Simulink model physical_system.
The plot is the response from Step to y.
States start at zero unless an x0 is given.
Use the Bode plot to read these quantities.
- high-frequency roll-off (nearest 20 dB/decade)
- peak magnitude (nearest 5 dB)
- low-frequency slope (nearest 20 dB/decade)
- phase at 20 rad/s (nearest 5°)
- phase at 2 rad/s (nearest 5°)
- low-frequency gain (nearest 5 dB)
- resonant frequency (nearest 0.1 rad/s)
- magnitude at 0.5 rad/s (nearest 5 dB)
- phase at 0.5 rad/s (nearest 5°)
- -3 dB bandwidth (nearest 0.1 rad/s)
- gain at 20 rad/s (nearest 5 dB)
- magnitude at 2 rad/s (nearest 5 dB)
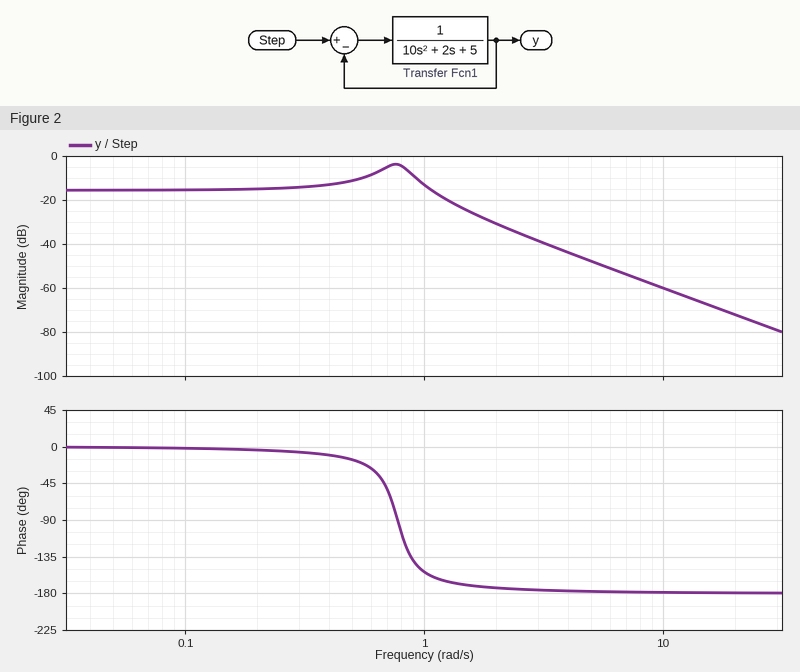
-40 dB/decade
-5 dB
0 dB/decade
-180°
-175°
-15 dB
0.8 rad/s
-10 dB
-15°
1.2 rad/s
-70 dB
-30 dB
